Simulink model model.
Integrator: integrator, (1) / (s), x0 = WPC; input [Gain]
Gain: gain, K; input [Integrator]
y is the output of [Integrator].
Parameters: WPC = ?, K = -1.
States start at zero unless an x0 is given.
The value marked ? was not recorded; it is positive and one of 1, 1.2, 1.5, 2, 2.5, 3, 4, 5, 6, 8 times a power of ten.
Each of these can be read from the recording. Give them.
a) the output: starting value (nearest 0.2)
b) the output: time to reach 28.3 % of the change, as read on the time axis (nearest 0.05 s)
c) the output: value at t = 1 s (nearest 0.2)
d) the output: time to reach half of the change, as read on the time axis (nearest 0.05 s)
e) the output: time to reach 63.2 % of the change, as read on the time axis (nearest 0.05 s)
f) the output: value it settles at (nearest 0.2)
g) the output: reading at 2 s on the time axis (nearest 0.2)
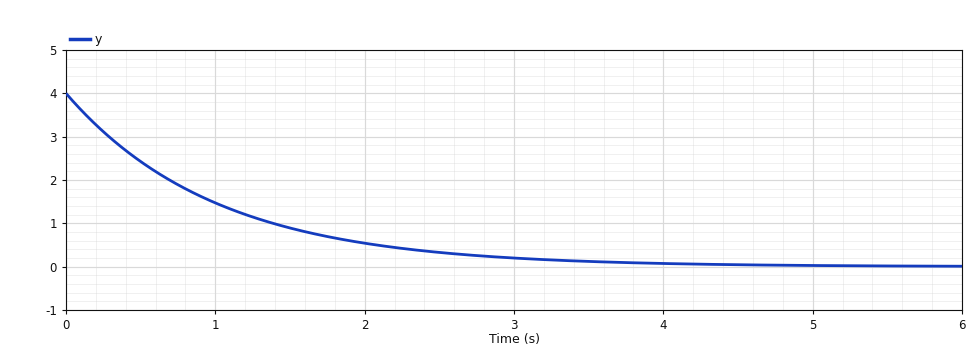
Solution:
4.0
0.35 s
1.4
0.70 s
1.00 s
0.0
0.6
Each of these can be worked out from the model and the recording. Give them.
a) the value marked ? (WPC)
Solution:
4
